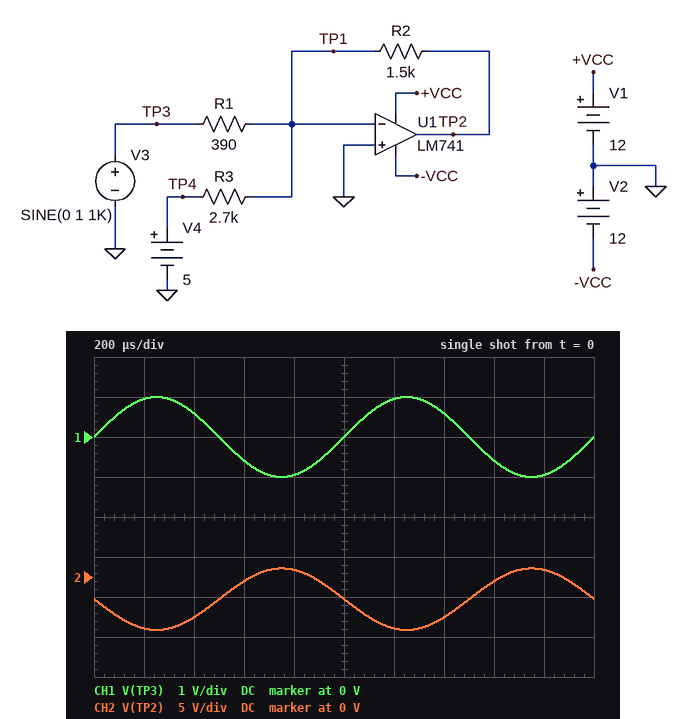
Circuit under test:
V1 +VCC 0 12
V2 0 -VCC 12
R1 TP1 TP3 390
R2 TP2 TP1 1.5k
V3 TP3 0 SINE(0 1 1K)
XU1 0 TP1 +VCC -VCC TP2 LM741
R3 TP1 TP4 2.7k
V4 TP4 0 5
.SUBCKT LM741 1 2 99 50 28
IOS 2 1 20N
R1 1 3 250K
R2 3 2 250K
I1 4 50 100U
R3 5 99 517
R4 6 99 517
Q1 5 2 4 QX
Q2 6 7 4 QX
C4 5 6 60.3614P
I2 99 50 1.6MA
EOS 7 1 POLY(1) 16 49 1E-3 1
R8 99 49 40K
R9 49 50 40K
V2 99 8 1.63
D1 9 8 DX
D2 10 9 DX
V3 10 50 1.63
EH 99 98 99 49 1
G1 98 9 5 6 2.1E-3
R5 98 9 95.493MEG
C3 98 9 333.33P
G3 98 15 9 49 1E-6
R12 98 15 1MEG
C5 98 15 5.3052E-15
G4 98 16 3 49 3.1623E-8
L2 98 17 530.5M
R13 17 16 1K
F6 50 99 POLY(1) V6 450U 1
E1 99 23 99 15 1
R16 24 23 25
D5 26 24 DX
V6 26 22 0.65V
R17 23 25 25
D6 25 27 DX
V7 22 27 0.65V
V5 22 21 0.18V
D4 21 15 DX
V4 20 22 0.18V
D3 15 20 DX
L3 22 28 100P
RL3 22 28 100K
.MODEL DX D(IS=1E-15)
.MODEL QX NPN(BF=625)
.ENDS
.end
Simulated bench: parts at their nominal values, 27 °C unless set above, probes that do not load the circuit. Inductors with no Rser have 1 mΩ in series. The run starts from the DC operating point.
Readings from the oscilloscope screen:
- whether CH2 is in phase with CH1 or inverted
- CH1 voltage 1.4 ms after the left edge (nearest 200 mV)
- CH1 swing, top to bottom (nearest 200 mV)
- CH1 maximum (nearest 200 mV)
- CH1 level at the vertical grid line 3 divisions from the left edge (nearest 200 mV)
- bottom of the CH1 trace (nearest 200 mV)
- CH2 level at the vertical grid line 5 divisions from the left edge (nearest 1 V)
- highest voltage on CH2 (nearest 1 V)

inverted
600 mV
2.0 V
1.0 V
-600 mV
-1.0 V
-3 V
1 V
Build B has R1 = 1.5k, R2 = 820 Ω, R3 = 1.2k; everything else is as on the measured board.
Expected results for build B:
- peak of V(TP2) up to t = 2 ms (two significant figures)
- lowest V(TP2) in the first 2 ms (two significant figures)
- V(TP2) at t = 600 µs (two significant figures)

-2.9 V
-4.0 V
-3.1 V
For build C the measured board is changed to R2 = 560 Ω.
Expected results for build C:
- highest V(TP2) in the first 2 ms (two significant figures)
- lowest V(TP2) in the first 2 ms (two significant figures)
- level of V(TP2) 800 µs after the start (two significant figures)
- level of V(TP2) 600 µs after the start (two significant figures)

400 mV
-2.5 V
330 mV
-190 mV
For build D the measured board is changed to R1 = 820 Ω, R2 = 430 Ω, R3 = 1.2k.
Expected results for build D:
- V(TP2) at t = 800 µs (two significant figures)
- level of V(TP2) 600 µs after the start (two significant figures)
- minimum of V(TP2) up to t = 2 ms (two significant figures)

-1.3 V
-1.5 V
-2.3 V
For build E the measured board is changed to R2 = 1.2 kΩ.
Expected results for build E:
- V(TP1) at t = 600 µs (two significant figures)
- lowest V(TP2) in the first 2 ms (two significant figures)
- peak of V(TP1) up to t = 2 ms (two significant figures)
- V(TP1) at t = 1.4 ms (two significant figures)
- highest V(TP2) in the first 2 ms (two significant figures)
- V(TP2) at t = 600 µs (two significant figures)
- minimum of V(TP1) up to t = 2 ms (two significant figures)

-1.7 mV
-5.3 V
4.2 mV
-1.5 mV
860 mV
-420 mV
-2.2 mV
